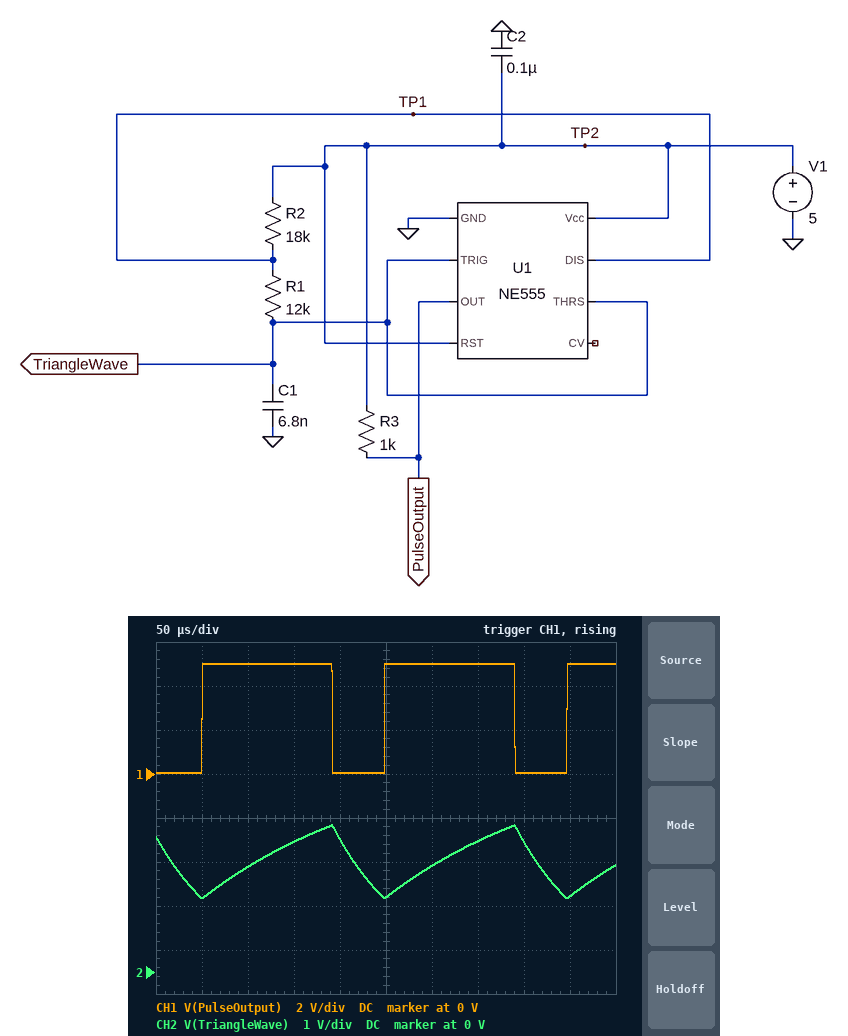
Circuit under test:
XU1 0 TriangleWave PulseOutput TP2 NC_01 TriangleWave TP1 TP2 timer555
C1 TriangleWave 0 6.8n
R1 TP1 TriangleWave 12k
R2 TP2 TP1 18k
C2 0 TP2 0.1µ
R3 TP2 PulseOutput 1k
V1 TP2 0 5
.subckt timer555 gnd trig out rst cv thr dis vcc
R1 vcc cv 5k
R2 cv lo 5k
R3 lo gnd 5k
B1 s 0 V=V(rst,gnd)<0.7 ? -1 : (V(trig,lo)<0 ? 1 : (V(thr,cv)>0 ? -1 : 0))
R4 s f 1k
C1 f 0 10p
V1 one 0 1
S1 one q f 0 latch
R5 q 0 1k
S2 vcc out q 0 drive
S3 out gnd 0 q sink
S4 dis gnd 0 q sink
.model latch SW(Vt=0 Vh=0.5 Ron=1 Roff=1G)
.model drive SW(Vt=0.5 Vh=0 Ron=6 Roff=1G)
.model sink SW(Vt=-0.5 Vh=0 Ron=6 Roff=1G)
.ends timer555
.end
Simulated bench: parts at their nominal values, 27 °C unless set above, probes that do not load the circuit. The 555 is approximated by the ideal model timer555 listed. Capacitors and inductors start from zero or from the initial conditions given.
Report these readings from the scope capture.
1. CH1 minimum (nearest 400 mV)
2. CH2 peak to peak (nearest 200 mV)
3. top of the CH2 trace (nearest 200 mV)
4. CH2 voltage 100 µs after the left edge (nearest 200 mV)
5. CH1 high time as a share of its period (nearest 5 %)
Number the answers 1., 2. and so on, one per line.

1. 0 V
2. 1.6 V
3. 3.4 V
4. 2.4 V
5. 70 %
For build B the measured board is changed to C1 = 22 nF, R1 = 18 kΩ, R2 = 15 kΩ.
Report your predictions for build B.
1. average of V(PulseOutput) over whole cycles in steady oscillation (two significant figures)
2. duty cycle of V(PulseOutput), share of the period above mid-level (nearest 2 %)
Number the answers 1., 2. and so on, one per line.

1. 3.2 V
2. 64 %
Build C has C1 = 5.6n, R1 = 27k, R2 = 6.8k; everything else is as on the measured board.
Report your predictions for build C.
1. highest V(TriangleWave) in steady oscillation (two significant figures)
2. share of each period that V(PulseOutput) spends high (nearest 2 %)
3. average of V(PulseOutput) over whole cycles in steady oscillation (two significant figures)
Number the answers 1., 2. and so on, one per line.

1. 3.3 V
2. 56 %
3. 2.8 V
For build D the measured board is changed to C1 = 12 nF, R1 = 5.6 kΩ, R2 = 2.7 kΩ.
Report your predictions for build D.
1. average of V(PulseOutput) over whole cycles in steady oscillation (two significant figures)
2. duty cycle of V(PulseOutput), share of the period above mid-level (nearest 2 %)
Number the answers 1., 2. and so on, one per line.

1. 3.0 V
2. 60 %
